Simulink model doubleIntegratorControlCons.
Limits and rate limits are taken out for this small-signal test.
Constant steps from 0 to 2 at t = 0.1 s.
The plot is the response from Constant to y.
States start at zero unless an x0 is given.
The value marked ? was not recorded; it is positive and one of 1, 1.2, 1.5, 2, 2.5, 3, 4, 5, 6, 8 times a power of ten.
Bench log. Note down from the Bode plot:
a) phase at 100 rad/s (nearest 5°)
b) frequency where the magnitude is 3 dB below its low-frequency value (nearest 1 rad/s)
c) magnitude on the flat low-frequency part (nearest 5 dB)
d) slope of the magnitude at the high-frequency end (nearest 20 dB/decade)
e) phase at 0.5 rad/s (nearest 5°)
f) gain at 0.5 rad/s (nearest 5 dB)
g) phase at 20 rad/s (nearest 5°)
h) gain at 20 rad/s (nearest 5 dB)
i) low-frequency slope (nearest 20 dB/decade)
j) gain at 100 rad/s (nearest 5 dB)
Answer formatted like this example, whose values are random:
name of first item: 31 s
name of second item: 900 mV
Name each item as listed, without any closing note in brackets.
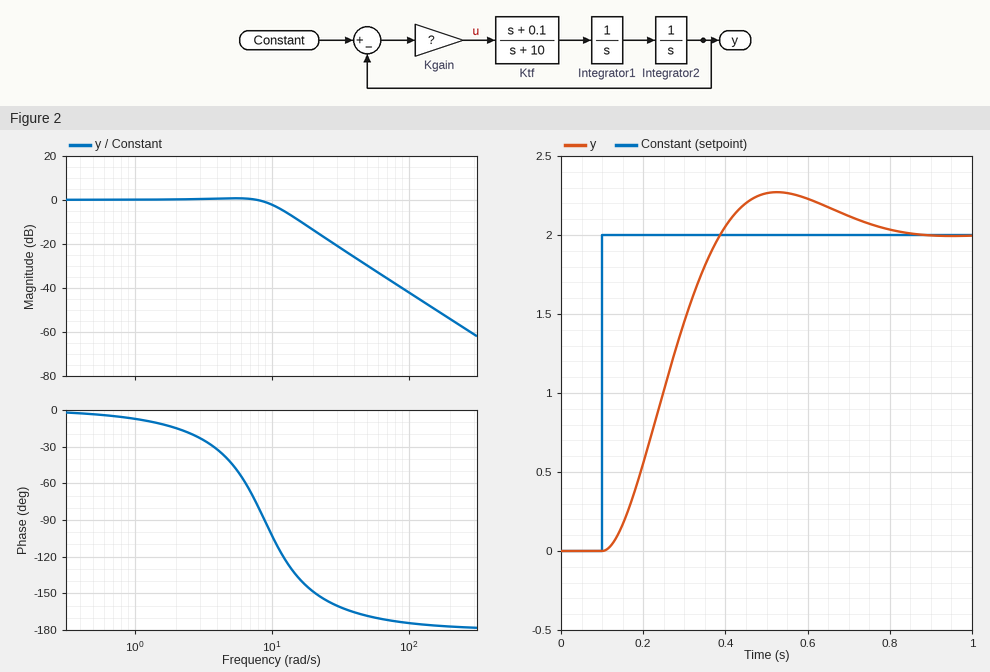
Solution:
phase at 100 rad/s: -175°
frequency where the magnitude is 3 dB below its low-frequency value: 11 rad/s
magnitude on the flat low-frequency part: 0 dB
slope of the magnitude at the high-frequency end: -40 dB/decade
phase at 0.5 rad/s: -5°
gain at 0.5 rad/s: 0 dB
phase at 20 rad/s: -150°
gain at 20 rad/s: -15 dB
low-frequency slope: 0 dB/decade
gain at 100 rad/s: -40 dB
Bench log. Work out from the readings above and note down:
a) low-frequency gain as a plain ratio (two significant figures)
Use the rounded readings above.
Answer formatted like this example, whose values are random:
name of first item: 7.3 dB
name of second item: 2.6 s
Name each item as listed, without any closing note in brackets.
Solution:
low-frequency gain as a plain ratio: 1.0
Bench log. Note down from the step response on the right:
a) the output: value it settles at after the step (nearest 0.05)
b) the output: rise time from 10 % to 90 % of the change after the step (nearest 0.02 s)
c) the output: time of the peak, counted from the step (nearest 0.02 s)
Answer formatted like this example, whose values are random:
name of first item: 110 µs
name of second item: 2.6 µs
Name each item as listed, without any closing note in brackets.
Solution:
the output: value it settles at after the step: 2.00
the output: rise time from 10 % to 90 % of the change after the step: 0.20 s
the output: time of the peak, counted from the step: 0.42 s
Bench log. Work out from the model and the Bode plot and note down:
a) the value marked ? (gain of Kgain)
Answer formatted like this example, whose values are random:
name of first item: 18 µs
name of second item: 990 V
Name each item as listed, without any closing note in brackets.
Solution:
the value marked ?: 80
